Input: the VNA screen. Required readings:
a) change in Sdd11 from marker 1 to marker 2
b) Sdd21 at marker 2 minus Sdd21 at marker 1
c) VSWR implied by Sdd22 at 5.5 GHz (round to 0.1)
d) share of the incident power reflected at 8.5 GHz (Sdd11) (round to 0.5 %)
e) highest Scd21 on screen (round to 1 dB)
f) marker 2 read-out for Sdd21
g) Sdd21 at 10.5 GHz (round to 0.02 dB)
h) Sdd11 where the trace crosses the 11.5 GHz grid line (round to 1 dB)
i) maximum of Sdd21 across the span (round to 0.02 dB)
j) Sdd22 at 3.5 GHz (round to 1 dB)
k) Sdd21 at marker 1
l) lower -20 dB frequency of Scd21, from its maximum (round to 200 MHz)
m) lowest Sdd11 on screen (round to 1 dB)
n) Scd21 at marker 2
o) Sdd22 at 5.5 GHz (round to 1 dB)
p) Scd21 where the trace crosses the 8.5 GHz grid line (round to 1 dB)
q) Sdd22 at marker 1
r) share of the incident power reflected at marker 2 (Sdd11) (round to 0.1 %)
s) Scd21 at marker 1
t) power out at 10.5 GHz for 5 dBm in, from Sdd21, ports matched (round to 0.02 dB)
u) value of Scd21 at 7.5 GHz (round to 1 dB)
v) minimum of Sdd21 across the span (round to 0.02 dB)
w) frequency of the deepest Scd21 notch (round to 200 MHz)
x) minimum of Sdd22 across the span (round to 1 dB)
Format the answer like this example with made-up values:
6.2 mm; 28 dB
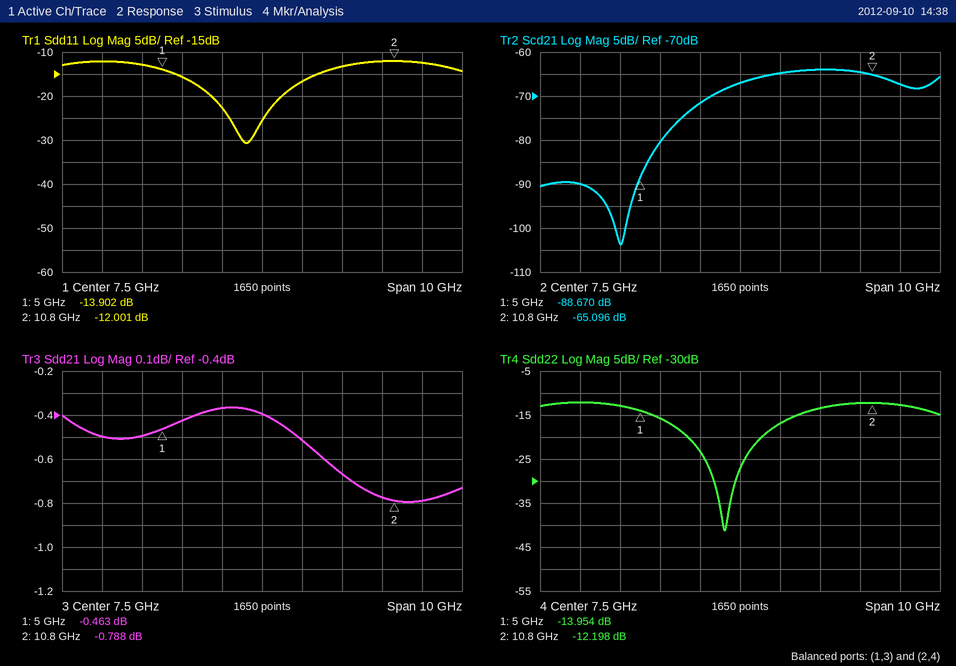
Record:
1.901 dB; -0.325 dB; 1.4; 2.0 %; -64 dB; -0.788 dB; -0.78 dB; -12 dB; -0.36 dB; -12 dB; -0.463 dB; 5.2 GHz; -31 dB; -65.096 dB; -16 dB; -65 dB; -13.954 dB; 6.3 %; -88.670 dB; 4.22 dBm; -67 dB; -0.80 dB; 4.6 GHz; -41 dB
